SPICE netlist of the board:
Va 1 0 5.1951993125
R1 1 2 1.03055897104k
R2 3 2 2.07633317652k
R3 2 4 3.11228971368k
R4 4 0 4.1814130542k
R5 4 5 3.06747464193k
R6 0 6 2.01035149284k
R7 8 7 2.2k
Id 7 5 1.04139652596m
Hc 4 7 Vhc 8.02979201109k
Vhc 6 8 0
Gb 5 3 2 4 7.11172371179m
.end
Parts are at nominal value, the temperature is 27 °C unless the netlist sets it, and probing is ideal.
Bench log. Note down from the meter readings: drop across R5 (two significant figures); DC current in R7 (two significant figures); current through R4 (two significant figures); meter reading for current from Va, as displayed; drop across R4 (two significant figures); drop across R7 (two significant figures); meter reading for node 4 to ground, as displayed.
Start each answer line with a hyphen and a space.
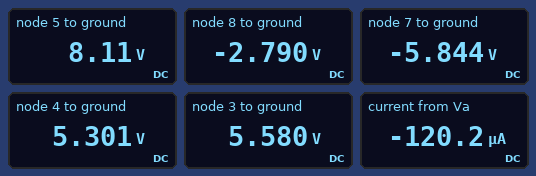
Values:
- 2.8 V
- 1.4 mA
- 1.3 mA
- -120.2 µA
- 5.3 V
- 3.1 V
- 5.301 V
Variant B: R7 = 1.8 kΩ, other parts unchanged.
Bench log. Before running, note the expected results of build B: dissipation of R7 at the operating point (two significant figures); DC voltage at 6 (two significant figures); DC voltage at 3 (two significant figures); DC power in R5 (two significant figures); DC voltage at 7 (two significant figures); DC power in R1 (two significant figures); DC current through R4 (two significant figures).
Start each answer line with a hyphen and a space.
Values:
- 2.7 mW
- -2.5 V
- 5.2 V
- 3.4 mW
- -4.7 V
- 130 nW
- 1.2 mA
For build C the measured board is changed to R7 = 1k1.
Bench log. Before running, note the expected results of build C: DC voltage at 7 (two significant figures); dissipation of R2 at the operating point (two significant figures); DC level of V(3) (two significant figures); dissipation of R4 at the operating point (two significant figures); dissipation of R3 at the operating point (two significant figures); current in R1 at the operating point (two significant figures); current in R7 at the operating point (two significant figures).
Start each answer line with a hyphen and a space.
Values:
- -3.2 V
- 74 µW
- 4.6 V
- 6.1 mW
- 230 nW
- 180 µA
- 1.0 mA
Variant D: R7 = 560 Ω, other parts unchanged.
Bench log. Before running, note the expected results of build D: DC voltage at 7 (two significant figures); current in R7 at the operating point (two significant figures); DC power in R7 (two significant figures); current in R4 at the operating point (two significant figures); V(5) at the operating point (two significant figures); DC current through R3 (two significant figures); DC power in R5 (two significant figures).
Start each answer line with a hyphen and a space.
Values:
- -2.3 V
- 910 µA
- 460 µW
- 1.2 mA
- 9.0 V
- 13 µA
- 5.4 mW
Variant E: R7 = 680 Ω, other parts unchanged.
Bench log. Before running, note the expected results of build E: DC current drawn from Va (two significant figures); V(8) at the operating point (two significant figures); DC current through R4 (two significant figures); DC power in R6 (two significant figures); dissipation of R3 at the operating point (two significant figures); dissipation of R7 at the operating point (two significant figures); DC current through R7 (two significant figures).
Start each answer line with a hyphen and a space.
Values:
- 260 µA
- -1.9 V
- 1.2 mA
- 1.7 mW
- 460 nW
- 590 µW
- 930 µA
